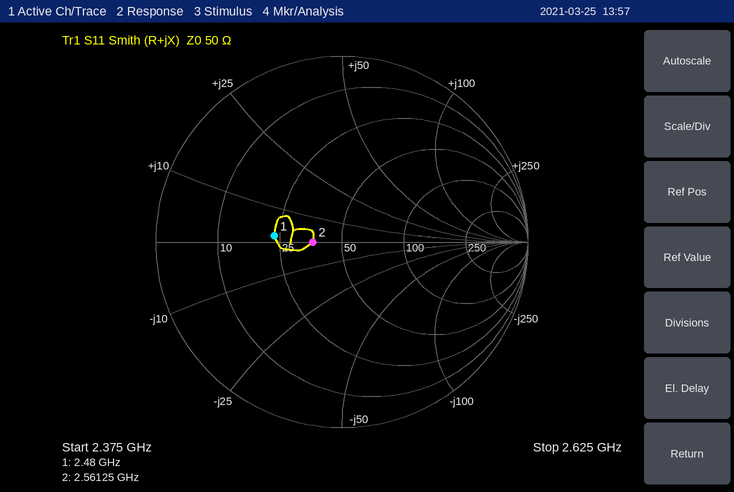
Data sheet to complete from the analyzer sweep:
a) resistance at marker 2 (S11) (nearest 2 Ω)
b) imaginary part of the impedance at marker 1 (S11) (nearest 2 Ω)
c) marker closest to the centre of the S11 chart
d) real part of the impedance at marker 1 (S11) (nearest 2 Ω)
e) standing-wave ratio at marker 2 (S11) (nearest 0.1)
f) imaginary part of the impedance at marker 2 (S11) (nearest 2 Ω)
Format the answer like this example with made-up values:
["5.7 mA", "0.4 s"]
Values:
["36 Ω", "+2 Ω", "marker 2", "24 Ω", "1.4", "0 Ω"]
